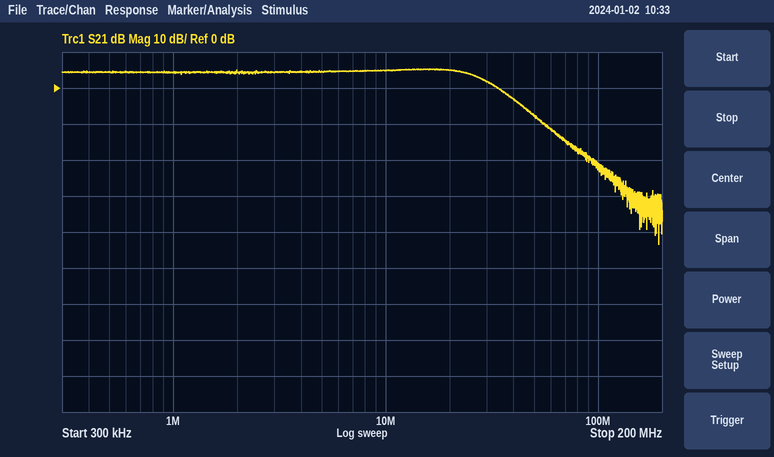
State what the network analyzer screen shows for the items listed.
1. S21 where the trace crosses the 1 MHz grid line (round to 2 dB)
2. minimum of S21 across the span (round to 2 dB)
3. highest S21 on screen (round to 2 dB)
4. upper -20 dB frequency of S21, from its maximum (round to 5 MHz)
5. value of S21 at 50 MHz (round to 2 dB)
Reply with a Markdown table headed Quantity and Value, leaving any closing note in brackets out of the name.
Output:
| Quantity | Value |
|---|---|
| S21 where the trace crosses the 1 MHz grid line | 4 dB |
| minimum of S21 across the span | -44 dB |
| highest S21 on screen | 6 dB |
| upper -20 dB frequency of S21, from its maximum | 70 MHz |
| value of S21 at 50 MHz | -8 dB |
